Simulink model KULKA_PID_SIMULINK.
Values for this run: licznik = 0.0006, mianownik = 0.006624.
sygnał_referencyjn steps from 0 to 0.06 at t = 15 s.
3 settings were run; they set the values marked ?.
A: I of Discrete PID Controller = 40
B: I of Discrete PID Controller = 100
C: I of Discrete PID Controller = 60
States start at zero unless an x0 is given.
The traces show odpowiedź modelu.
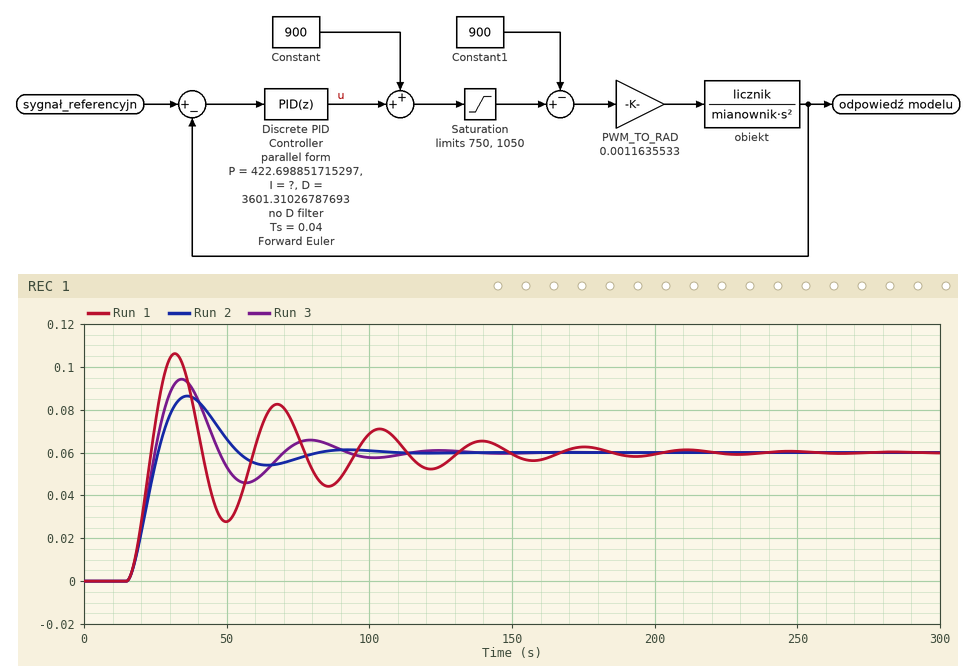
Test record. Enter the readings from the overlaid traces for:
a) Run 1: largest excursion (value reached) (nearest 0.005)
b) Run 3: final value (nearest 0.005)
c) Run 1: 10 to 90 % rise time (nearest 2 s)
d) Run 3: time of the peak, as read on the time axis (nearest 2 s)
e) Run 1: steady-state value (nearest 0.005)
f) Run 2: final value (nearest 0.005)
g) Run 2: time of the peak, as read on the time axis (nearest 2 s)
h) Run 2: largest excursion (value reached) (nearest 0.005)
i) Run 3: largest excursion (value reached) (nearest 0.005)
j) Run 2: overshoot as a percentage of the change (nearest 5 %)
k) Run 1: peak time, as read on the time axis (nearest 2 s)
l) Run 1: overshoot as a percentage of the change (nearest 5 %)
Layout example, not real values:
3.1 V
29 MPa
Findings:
0.105
0.060
6 s
34 s
0.060
0.060
36 s
0.085
0.095
45 %
32 s
75 %
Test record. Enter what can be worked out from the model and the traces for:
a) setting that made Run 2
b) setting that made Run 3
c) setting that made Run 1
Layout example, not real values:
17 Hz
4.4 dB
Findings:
A
C
B
